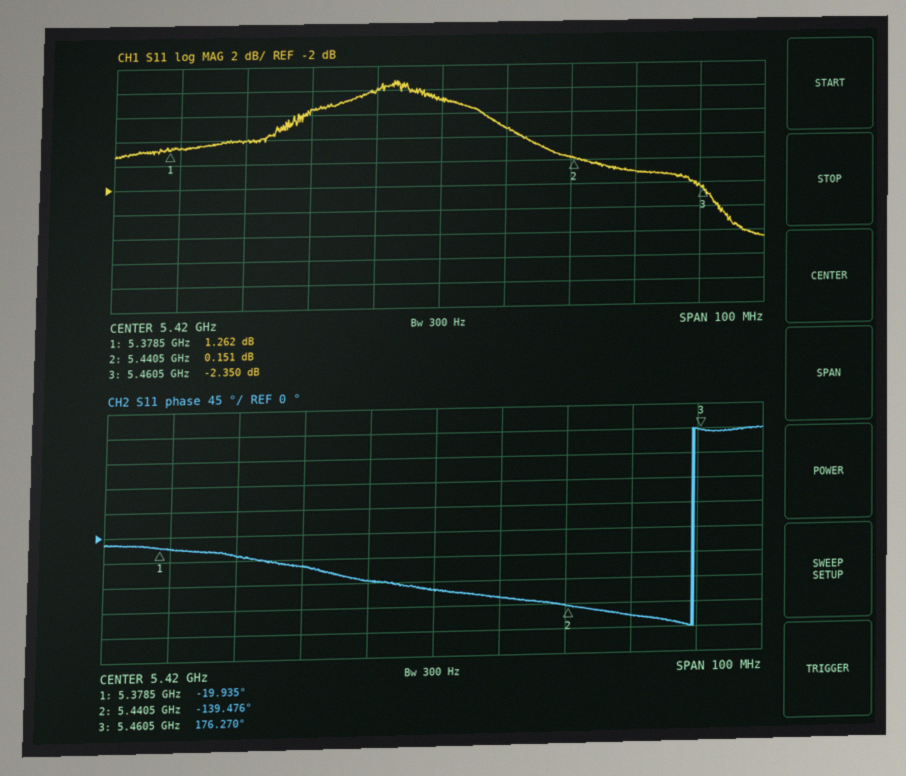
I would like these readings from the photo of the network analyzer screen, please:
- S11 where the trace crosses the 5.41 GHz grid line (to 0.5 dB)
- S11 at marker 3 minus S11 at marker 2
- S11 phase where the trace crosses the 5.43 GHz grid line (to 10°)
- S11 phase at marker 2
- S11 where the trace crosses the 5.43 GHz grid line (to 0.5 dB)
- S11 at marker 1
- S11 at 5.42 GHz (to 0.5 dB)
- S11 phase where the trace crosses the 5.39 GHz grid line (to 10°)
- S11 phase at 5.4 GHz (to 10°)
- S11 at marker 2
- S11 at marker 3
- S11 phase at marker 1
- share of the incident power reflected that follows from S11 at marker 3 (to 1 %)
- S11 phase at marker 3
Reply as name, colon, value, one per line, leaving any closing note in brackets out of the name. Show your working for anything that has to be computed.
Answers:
S11 where the trace crosses the 5.41 GHz grid line: 6.0 dB
S11 at marker 3 minus S11 at marker 2: -2.35 − (0.151) = -2.501 dB
S11 phase where the trace crosses the 5.43 GHz grid line: -120°
S11 phase at marker 2: -139.476°
S11 where the trace crosses the 5.43 GHz grid line: 2.5 dB
S11 at marker 1: 1.262 dB
S11 at 5.42 GHz: 5.0 dB
S11 phase where the trace crosses the 5.39 GHz grid line: -40°
S11 phase at 5.4 GHz: -60°
S11 at marker 2: 0.151 dB
S11 at marker 3: -2.350 dB
S11 phase at marker 1: -19.935°
share of the incident power reflected that follows from S11 at marker 3: 10^(-2.35/10) ≈ 58 %
S11 phase at marker 3: 176.270°
